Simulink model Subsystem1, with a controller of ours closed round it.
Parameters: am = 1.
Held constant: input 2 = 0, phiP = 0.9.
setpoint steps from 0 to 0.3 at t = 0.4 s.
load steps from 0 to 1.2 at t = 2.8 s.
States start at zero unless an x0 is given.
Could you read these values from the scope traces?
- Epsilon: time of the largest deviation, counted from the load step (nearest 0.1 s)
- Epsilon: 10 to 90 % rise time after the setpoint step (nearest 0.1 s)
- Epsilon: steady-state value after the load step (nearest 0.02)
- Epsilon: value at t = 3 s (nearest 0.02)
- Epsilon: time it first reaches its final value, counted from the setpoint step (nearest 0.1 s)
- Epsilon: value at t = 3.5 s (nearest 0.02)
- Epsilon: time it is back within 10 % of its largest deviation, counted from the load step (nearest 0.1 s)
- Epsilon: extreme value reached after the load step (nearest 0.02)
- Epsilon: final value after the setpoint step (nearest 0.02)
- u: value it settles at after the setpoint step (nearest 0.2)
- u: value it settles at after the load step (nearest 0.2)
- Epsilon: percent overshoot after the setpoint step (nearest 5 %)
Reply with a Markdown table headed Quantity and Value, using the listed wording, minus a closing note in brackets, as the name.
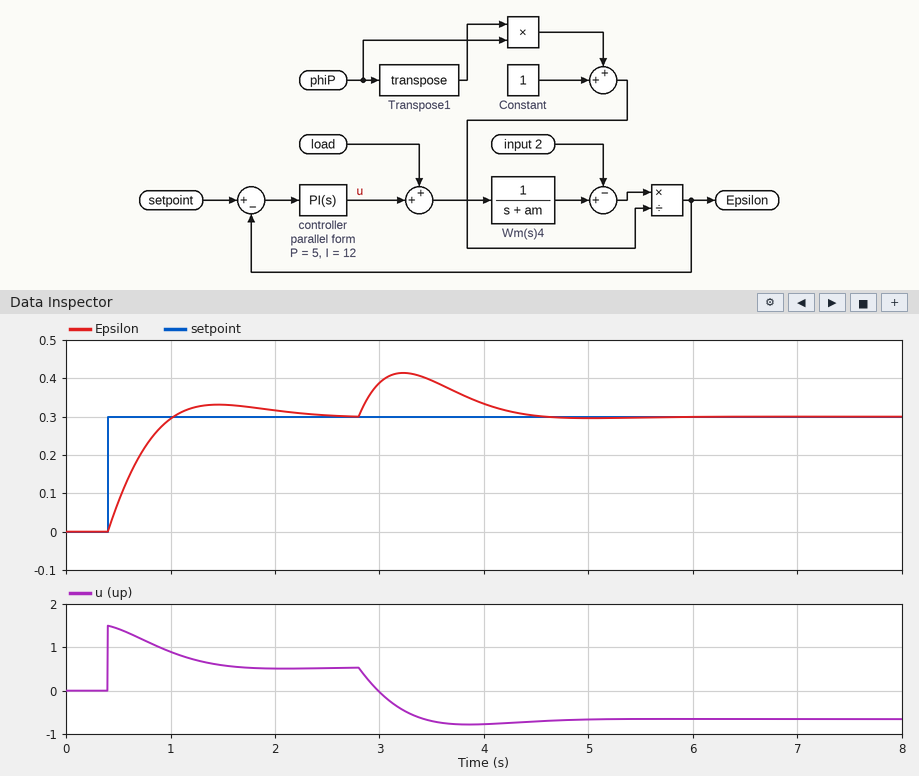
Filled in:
| Quantity | Value |
|---|---|
| Epsilon: time of the largest deviation, counted from the load step | 0.4 s |
| Epsilon: 10 to 90 % rise time after the setpoint step | 0.5 s |
| Epsilon: steady-state value after the load step | 0.30 |
| Epsilon: value at t = 3 s | 0.38 |
| Epsilon: time it first reaches its final value, counted from the setpoint step | 0.6 s |
| Epsilon: value at t = 3.5 s | 0.40 |
| Epsilon: time it is back within 10 % of its largest deviation, counted from the load step | 1.5 s |
| Epsilon: extreme value reached after the load step | 0.42 |
| Epsilon: final value after the setpoint step | 0.30 |
| u: value it settles at after the setpoint step | 0.6 |
| u: value it settles at after the load step | -0.6 |
| Epsilon: percent overshoot after the setpoint step | 10 % |
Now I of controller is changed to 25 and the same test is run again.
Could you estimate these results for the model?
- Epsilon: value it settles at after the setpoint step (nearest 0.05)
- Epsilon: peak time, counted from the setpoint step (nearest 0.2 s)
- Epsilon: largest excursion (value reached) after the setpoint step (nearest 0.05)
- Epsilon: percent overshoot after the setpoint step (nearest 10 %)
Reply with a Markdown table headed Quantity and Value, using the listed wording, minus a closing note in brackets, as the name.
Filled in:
| Quantity | Value |
|---|---|
| Epsilon: value it settles at after the setpoint step | 0.30 |
| Epsilon: peak time, counted from the setpoint step | 0.8 s |
| Epsilon: largest excursion (value reached) after the setpoint step | 0.35 |
| Epsilon: percent overshoot after the setpoint step | 20 % |
